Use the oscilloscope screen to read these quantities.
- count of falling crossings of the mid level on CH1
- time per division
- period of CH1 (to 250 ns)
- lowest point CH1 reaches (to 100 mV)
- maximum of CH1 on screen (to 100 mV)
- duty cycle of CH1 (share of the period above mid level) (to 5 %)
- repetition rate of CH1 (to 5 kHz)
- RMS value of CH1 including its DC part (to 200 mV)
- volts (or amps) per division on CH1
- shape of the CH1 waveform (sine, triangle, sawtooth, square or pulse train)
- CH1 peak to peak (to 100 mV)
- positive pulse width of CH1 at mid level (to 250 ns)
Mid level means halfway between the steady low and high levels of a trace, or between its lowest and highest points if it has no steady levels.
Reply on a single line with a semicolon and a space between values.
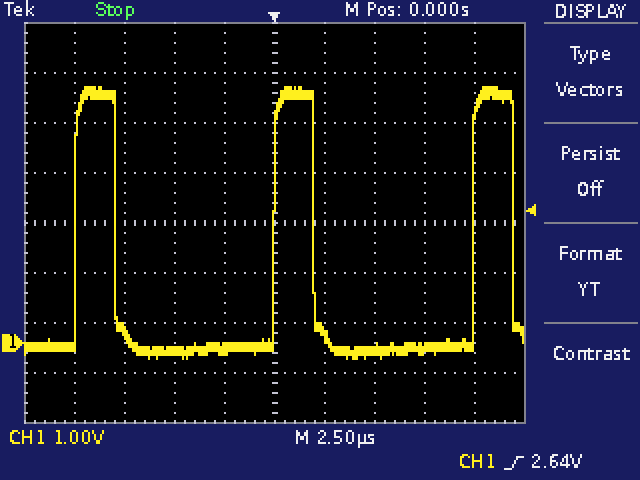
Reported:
3; 2.5 µs; 10.00 µs; -300 mV; 5.1 V; 20 %; 100 kHz; 2.2 V; 1 V; pulse train; 5.4 V; 2.00 µs
